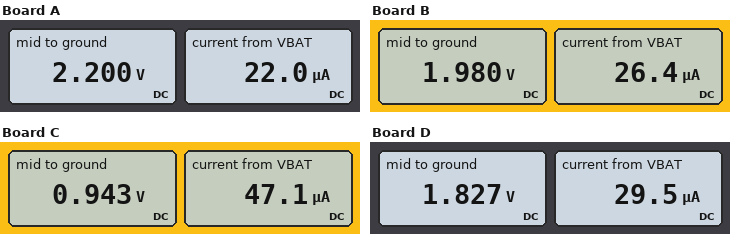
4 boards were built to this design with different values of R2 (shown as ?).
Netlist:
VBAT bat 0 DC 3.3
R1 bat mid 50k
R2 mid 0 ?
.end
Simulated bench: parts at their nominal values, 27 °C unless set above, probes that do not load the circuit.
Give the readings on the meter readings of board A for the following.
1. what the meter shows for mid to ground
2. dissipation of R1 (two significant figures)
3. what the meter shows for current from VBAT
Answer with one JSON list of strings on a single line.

["2.200 V", "24 µW", "22.0 µA"]
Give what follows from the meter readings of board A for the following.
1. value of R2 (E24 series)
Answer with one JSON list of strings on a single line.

["100 kΩ"]
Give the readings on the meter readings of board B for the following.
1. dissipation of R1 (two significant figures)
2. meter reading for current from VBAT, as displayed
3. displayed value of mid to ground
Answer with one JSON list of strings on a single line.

["35 µW", "26.4 µA", "1.980 V"]
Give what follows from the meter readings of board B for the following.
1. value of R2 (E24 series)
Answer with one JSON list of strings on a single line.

["75 kΩ"]
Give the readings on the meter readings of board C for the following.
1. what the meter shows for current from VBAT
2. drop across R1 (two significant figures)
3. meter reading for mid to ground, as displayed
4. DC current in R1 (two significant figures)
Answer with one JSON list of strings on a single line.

["47.1 µA", "2.4 V", "0.943 V", "47 µA"]
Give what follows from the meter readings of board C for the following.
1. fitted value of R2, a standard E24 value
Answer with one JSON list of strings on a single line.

["20 kΩ"]
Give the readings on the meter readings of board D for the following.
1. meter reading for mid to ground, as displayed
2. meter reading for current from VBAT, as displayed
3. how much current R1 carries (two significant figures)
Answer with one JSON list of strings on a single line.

["1.827 V", "29.5 µA", "29 µA"]
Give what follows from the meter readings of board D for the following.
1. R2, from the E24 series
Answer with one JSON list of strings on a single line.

["62 kΩ"]
